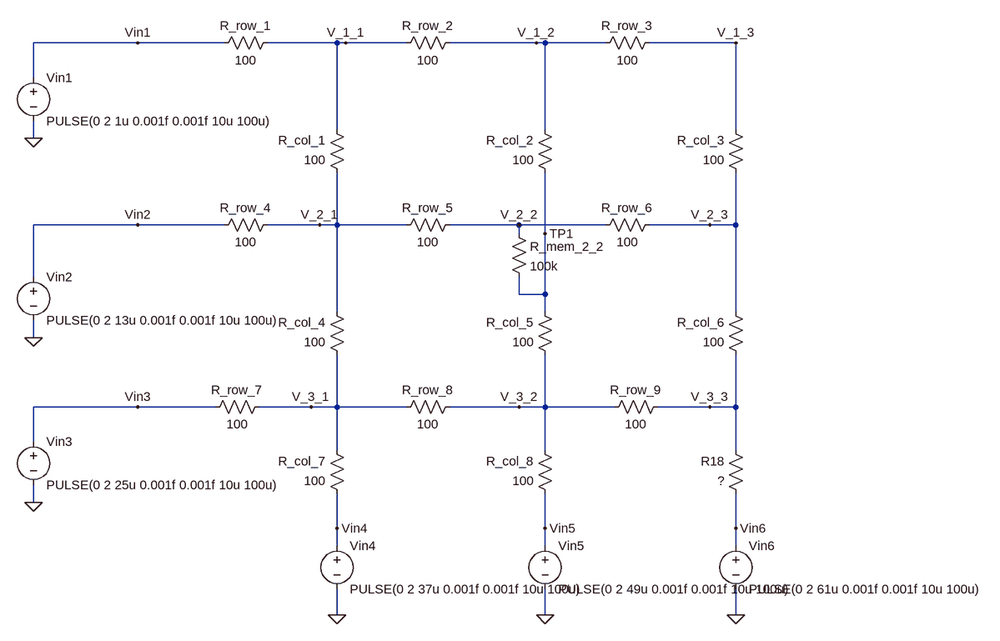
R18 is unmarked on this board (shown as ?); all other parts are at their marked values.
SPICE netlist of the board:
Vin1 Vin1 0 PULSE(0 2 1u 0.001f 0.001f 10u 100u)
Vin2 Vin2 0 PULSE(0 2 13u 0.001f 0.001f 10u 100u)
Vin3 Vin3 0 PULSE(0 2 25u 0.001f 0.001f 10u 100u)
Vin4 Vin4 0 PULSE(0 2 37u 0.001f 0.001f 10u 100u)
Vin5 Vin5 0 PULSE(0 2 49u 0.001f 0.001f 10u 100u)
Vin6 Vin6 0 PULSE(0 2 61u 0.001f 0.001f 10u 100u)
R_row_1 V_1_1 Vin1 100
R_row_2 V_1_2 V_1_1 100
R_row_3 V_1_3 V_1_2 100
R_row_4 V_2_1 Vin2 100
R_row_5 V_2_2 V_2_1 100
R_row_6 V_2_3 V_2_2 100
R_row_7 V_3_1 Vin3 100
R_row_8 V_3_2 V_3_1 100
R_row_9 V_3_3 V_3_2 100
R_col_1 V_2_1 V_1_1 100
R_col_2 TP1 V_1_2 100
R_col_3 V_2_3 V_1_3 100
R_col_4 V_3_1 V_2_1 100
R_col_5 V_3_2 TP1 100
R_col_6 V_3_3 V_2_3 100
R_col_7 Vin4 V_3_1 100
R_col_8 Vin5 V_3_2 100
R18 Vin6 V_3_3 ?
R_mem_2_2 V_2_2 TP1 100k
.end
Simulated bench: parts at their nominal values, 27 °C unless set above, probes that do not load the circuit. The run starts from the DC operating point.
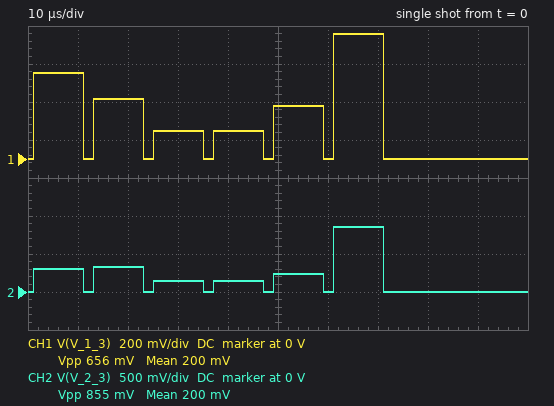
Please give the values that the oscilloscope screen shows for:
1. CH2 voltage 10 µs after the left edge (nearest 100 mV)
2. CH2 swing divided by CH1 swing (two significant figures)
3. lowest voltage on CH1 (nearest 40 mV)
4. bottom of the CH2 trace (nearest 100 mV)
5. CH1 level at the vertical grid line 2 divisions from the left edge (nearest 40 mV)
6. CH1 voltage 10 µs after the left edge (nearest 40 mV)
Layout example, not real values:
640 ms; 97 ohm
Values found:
300 mV; 1.3; 0 V; 0 V; 320 mV; 440 mV
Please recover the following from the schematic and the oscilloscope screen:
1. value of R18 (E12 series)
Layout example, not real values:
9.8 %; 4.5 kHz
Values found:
47 Ω
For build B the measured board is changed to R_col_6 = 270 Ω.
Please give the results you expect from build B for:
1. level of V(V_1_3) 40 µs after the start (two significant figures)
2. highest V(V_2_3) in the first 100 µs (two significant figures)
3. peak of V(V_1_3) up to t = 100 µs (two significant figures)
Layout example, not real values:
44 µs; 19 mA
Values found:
170 mV; 590 mV; 520 mV
